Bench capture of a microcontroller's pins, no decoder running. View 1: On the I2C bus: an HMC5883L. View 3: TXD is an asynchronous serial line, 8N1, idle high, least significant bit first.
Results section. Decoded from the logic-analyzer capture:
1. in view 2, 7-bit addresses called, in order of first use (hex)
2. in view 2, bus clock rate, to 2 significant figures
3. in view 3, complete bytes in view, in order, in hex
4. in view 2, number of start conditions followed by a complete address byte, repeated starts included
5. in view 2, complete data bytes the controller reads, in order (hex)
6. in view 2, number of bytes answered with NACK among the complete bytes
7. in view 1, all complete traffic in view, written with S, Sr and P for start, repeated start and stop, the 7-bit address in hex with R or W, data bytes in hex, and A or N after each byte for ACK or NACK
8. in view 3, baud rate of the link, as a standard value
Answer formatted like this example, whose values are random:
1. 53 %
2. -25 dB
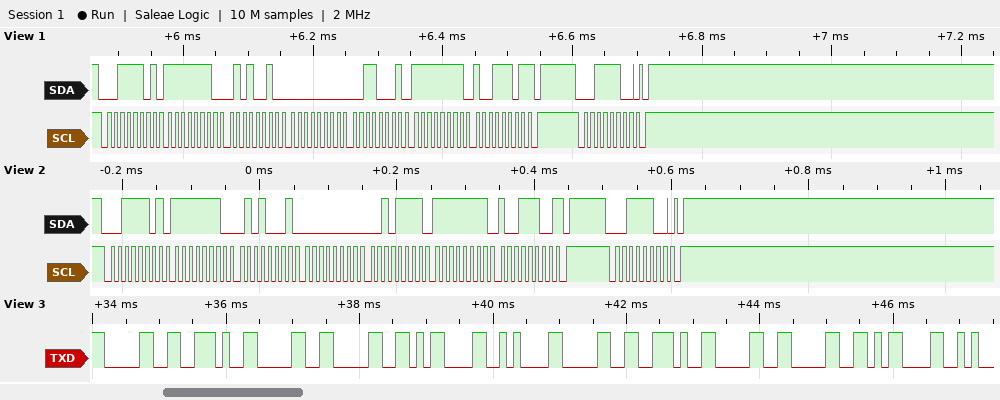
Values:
1. 0x1E
2. 100 kHz
3. 0x30 0x2E 0x30 0x30 0x0D 0x0A 0x30 0x2E 0x30 0x30 0x0D
4. 2
5. FE 51 00 2F FF 9C
6. 1
7. S 1ER A FE A 52 A 00 A 31 A FF A 9D N P S 1EW A P
8. 9600 baud
